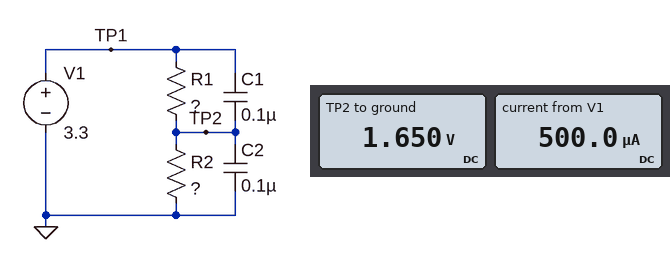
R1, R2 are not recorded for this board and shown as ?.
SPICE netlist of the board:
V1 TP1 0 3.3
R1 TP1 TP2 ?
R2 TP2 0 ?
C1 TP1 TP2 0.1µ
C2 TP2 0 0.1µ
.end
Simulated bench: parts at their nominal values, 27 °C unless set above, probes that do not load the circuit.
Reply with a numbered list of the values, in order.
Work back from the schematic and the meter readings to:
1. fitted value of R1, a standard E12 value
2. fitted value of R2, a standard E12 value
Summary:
1. 3.3 kΩ
2. 3.3 kΩ
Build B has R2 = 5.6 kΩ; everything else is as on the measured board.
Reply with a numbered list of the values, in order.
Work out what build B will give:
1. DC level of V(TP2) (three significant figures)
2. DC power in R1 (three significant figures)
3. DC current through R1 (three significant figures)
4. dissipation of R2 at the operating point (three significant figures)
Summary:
1. 2.08 V
2. 454 µW
3. 371 µA
4. 770 µW
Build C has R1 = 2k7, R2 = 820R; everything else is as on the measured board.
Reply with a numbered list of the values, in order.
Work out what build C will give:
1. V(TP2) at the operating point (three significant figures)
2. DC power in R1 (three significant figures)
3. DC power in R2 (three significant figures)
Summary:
1. 769 mV
2. 2.37 mW
3. 721 µW
